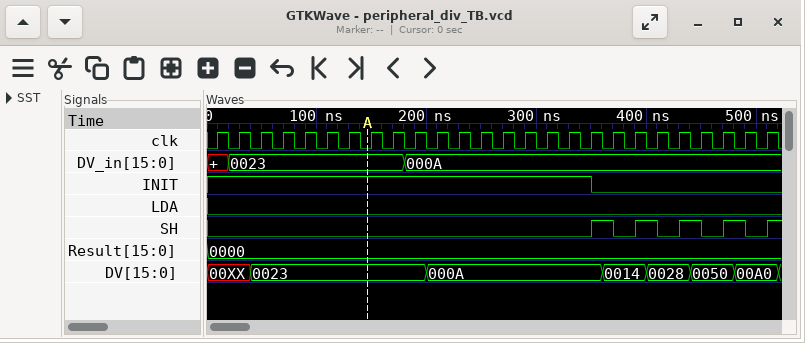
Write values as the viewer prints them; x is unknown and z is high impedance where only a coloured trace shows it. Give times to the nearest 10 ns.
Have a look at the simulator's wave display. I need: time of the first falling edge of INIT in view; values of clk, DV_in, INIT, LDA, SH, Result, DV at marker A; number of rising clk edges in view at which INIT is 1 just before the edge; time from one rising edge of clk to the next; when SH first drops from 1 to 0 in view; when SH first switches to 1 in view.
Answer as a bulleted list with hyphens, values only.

- 350 ns
- clk=0, DV_in=0023, INIT=1, LDA=0, SH=0, Result=0000, DV=0023
- 18
- 20 ns
- 370 ns
- 350 ns
